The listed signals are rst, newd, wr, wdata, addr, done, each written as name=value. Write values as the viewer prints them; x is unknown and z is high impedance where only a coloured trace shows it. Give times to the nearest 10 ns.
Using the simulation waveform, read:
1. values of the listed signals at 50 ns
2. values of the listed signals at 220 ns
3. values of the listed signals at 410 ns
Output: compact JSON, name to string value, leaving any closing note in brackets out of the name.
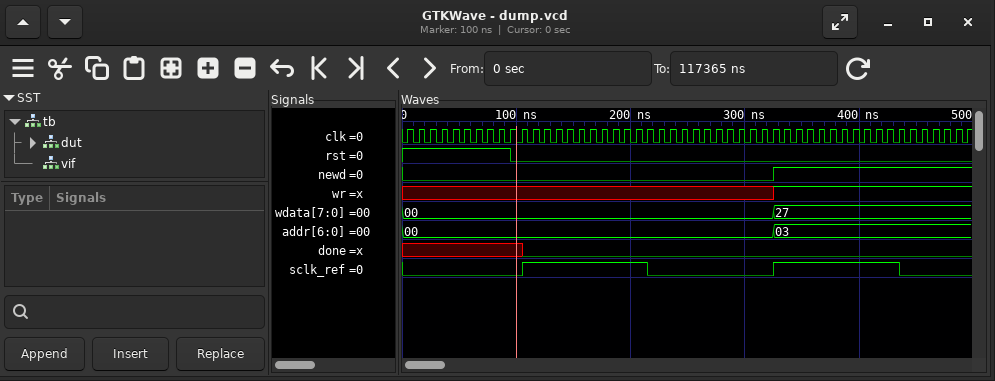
{"values of the listed signals at 50 ns": "rst=1, newd=0, wr=x, wdata=00, addr=00, done=x", "values of the listed signals at 220 ns": "rst=0, newd=0, wr=x, wdata=00, addr=00, done=0", "values of the listed signals at 410 ns": "rst=0, newd=1, wr=1, wdata=27, addr=03, done=0"}
